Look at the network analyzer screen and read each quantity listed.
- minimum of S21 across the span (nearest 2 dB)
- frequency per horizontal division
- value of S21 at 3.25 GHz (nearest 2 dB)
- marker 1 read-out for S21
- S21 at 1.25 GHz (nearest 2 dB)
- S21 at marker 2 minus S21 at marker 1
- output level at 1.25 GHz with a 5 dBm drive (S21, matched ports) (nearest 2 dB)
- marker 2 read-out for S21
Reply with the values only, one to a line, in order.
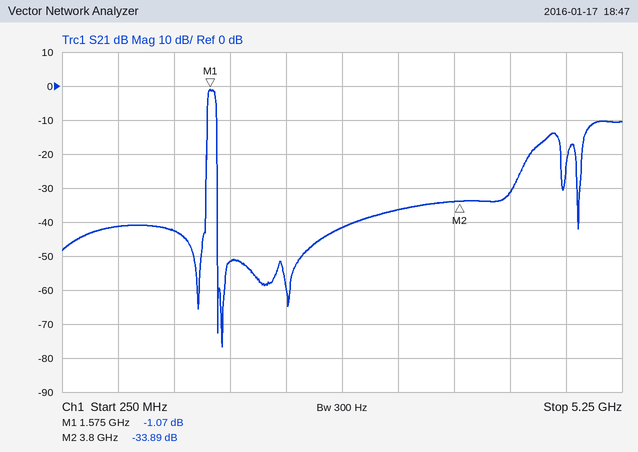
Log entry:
-76 dB
500 MHz
-36 dB
-1.07 dB
-42 dB
-32.82 dB
-38 dBm
-33.89 dB
